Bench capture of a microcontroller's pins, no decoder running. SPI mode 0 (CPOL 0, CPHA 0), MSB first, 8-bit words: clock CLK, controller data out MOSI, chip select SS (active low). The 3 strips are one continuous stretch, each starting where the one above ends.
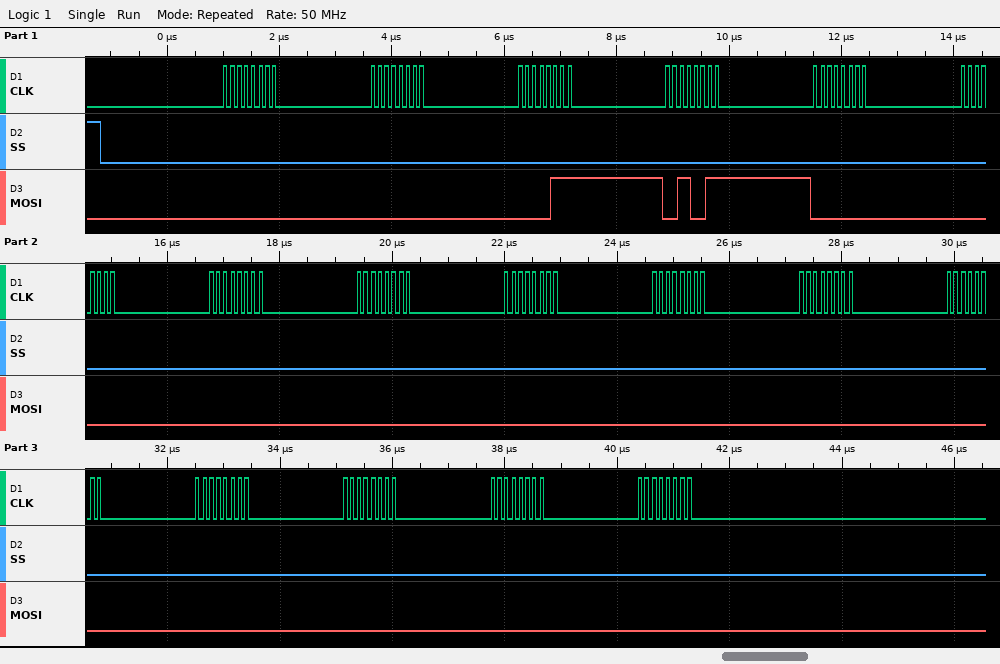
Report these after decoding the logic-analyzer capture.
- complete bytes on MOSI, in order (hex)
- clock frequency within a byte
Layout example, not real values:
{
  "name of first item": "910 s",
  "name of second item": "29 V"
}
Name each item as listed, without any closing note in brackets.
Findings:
{
  "complete bytes on MOSI, in order": "00 00 07 33 00 00 00 00 00 00 00 00 00 00 00 00",
  "clock frequency within a byte": "8 MHz"
}
